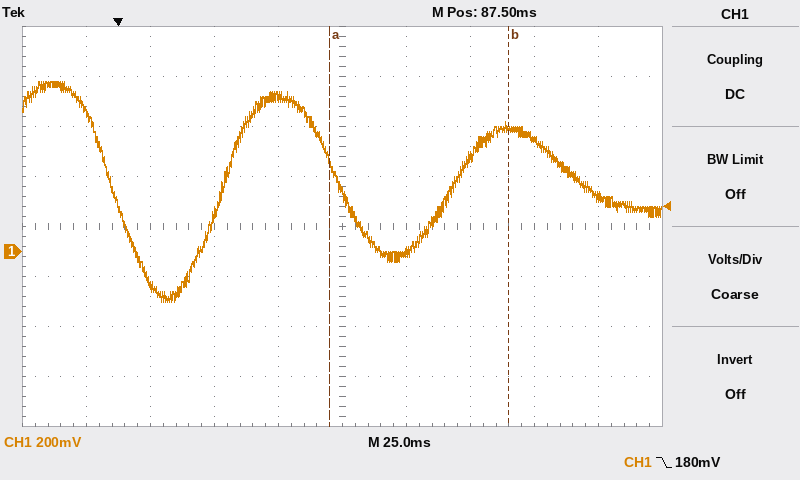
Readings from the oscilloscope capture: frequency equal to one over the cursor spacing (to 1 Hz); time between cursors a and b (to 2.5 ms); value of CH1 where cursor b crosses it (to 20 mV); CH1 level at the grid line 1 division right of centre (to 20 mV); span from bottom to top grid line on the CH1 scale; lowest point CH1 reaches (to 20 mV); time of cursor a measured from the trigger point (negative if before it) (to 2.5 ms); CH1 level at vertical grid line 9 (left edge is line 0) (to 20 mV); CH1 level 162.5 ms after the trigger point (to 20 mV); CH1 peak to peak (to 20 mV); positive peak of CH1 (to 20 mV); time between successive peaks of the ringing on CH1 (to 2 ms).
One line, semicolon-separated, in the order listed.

14 Hz; 70.0 ms; 500 mV; 0 mV; 1.6 V; -200 mV; +82.5 ms; 220 mV; 440 mV; 880 mV; 680 mV; 88 ms
